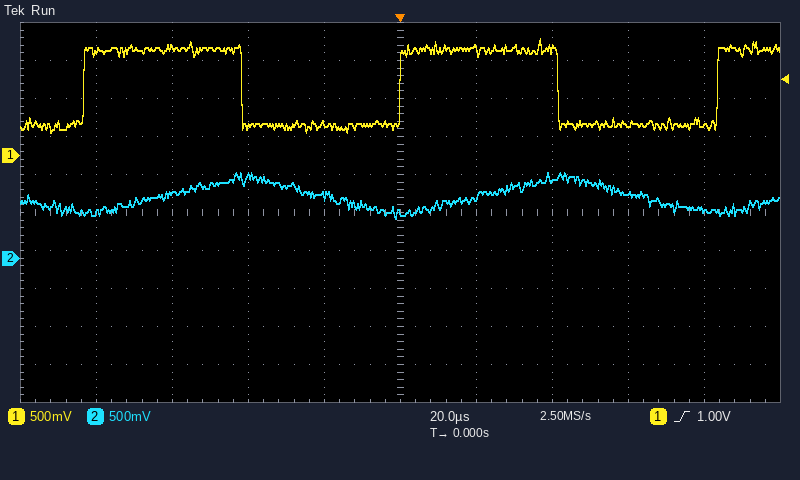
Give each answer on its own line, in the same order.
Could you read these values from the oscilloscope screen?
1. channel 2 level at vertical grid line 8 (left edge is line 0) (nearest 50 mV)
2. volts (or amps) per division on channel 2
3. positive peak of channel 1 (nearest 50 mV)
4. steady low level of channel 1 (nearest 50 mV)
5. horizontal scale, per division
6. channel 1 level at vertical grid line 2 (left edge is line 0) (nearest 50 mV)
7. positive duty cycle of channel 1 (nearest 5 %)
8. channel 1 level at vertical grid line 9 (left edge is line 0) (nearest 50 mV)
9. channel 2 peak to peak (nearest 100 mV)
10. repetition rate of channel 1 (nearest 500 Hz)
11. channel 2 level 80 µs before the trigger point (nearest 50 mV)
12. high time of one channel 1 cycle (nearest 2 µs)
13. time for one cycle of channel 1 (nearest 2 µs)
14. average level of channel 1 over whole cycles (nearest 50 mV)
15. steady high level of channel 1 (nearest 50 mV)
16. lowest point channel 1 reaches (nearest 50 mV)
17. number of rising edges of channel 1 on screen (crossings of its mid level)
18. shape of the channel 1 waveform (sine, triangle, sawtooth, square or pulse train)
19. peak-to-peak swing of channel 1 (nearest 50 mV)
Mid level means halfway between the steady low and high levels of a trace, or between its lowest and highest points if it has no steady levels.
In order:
850 mV
500 mV
1.55 V
400 mV
20 µs
1.40 V
50 %
400 mV
600 mV
12.0 kHz
600 mV
42 µs
84 µs
900 mV
1.40 V
300 mV
3
square
1.25 V
